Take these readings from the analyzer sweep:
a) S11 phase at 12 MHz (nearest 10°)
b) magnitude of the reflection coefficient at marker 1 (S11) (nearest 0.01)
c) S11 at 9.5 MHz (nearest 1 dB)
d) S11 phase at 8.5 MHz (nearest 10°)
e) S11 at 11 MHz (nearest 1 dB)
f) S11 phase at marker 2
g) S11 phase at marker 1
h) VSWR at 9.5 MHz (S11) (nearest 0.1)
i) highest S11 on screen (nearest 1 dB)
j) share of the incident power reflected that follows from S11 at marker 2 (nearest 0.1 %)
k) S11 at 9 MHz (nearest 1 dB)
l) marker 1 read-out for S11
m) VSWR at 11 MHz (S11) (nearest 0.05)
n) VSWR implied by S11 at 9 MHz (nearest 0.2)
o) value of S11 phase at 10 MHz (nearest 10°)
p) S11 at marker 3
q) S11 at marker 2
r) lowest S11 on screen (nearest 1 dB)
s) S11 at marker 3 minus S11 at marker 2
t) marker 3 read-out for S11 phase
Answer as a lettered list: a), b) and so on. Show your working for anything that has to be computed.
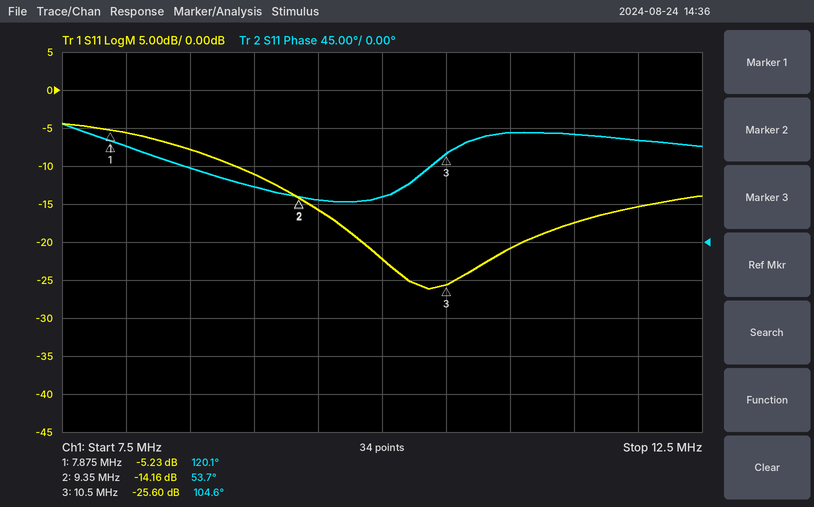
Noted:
a) 120°
b) 10^(-5.23/20) ≈ 0.55
c) -16 dB
d) 90°
e) -21 dB
f) 53.7°
g) 120.1°
h) |Γ| = 10^(-16/20) = 0.1585; VSWR = (1 + 0.1585)/(1 − 0.1585) ≈ 1.4
i) -4 dB
j) 10^(-14.16/10) ≈ 3.8 %
k) -11 dB
l) -5.23 dB
m) |Γ| = 10^(-21/20) = 0.0891; VSWR = (1 + 0.0891)/(1 − 0.0891) ≈ 1.20
n) |Γ| = 10^(-11/20) = 0.2818; VSWR = (1 + 0.2818)/(1 − 0.2818) ≈ 1.8
o) 50°
p) -25.60 dB
q) -14.16 dB
r) -26 dB
s) -25.6 − (-14.16) = -11.44 dB
t) 104.6°
